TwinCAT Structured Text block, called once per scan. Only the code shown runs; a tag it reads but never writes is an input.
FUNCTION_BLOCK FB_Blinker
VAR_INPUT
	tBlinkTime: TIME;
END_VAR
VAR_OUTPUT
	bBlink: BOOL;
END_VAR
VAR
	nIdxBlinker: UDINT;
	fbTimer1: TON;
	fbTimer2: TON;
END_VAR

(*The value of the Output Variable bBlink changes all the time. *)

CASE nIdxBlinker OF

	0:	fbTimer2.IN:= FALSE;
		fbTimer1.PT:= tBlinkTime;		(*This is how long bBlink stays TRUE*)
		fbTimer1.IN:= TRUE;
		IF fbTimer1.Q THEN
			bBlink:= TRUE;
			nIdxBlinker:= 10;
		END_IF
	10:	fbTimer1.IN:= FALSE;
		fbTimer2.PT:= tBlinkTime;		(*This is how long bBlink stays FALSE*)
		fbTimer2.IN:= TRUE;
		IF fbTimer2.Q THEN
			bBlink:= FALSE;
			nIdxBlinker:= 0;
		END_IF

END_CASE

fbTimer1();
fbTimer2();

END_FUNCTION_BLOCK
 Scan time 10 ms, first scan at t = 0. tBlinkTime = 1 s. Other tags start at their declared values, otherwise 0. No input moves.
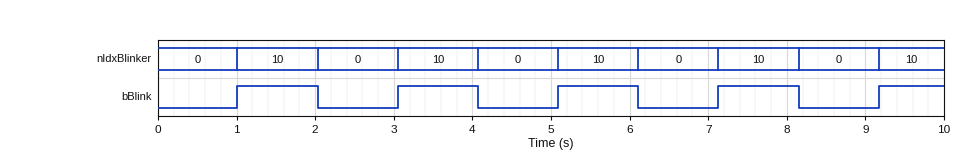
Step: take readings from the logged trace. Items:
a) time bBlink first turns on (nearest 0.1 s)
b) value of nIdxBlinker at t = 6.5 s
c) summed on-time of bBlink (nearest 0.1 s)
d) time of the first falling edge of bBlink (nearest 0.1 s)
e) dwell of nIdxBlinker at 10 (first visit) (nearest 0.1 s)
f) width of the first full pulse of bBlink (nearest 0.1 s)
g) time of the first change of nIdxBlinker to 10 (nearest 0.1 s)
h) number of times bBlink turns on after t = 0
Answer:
1.0 s
0
4.9 s
2.0 s
1.0 s
1.0 s
1.0 s
5
